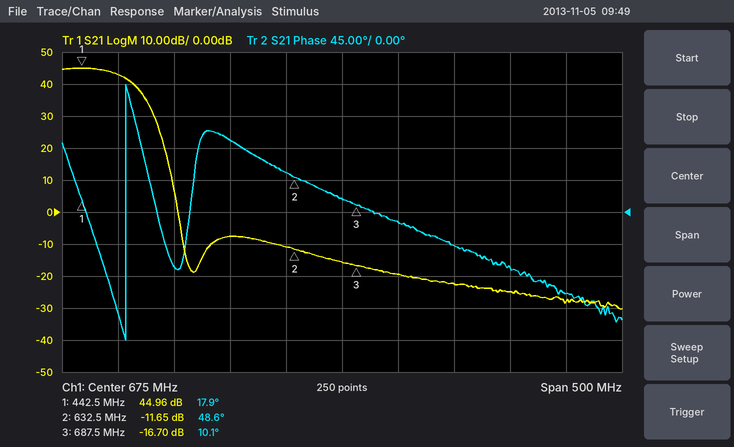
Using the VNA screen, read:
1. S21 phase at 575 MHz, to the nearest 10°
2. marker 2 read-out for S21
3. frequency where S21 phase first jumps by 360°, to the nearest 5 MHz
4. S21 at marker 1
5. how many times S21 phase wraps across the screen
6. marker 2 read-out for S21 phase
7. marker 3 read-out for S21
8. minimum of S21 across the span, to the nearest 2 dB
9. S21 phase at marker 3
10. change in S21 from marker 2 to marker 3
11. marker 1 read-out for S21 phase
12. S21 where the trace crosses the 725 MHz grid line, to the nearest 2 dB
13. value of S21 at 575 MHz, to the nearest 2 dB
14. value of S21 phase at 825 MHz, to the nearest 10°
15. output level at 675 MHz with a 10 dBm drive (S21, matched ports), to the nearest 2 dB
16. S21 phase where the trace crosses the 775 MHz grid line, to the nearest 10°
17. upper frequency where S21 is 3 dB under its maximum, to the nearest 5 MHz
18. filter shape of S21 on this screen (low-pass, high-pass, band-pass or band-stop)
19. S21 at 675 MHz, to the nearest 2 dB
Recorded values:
100°
-11.65 dB
480 MHz
44.96 dB
1
48.6°
-16.70 dB
-30 dB
10.1°
-5.05 dB
17.9°
-20 dB
-8 dB
-80°
-6 dBm
-50°
480 MHz
low-pass
-16 dB
